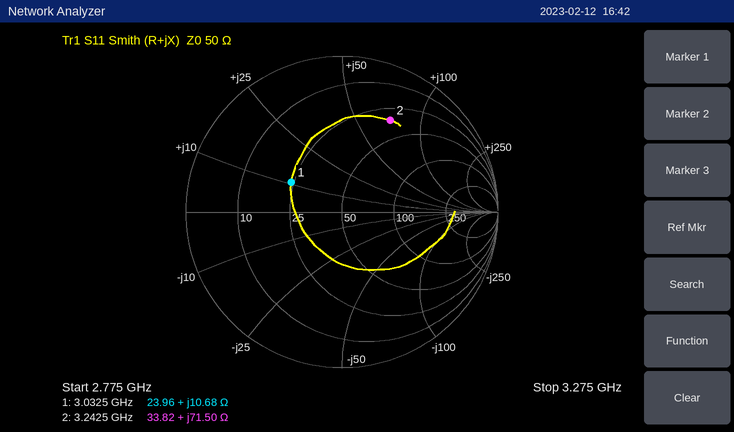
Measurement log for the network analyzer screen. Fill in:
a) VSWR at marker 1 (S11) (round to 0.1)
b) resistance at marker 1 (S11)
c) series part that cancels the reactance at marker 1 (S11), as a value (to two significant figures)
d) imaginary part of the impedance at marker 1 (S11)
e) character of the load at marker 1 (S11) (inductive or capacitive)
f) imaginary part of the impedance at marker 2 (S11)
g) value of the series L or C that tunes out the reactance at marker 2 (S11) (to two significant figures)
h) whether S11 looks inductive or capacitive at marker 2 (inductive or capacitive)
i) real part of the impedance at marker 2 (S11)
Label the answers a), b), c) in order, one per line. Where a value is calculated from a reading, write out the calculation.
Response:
a) 2.2
b) 23.96 Ω
c) C = 1/(2π × 3.0325 GHz × 10.68 Ω) ≈ 4.9 pF
d) +10.68 Ω
e) inductive
f) +71.50 Ω
g) C = 1/(2π × 3.2425 GHz × 71.5 Ω) ≈ 686 fF, so 690 fF to two significant figures
h) inductive
i) 33.82 Ω
